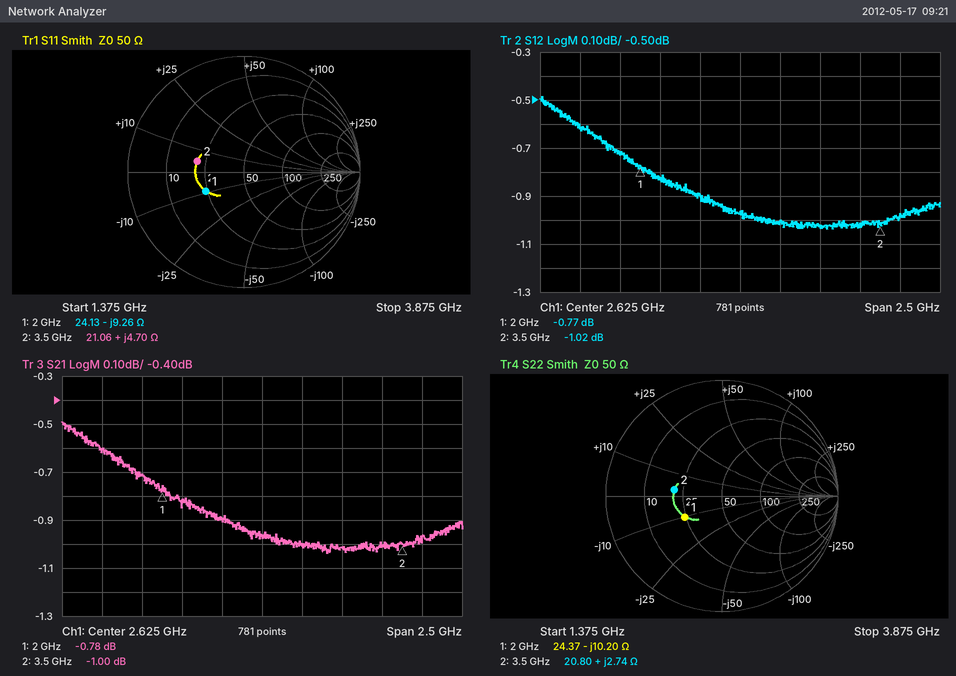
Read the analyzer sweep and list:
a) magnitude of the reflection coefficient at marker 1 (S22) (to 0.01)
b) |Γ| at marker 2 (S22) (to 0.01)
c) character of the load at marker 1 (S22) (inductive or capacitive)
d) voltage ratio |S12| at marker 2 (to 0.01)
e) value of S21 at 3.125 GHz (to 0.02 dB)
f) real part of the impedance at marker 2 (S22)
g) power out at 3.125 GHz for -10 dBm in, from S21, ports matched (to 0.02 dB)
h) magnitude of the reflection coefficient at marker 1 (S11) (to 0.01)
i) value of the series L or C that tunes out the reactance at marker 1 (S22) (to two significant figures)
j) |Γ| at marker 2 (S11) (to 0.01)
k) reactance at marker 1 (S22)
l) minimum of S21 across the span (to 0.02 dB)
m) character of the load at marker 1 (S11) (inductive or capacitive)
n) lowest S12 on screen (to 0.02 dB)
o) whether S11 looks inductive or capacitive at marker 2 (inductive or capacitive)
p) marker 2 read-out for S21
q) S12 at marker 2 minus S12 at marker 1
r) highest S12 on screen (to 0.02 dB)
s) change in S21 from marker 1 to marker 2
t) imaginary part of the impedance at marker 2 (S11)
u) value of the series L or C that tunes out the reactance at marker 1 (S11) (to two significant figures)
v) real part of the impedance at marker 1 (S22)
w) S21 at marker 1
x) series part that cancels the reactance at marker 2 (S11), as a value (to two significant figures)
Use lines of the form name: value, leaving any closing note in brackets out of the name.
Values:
magnitude of the reflection coefficient at marker 1 (S22): 0.37
|Γ| at marker 2 (S22): 0.41
character of the load at marker 1 (S22): capacitive
voltage ratio |S12| at marker 2: 0.89
value of S21 at 3.125 GHz: -1.02 dB
real part of the impedance at marker 2: 20.80 Ω
power out at 3.125 GHz for -10 dBm in, from S21, ports matched: -11.02 dBm
magnitude of the reflection coefficient at marker 1 (S11): 0.37
value of the series L or C that tunes out the reactance at marker 1 (S22): 810 pH
|Γ| at marker 2 (S11): 0.41
reactance at marker 1: -10.20 Ω
minimum of S21 across the span: -1.04 dB
character of the load at marker 1 (S11): capacitive
lowest S12 on screen: -1.04 dB
whether S11 looks inductive or capacitive at marker 2: inductive
marker 2 read-out for S21: -1.00 dB
S12 at marker 2 minus S12 at marker 1: -0.25 dB
highest S12 on screen: -0.48 dB
change in S21 from marker 1 to marker 2: -0.22 dB
imaginary part of the impedance at marker 2: +4.70 Ω
value of the series L or C that tunes out the reactance at marker 1 (S11): 740 pH
real part of the impedance at marker 1: 24.37 Ω
S21 at marker 1: -0.78 dB
series part that cancels the reactance at marker 2 (S11), as a value: 9.7 pF
